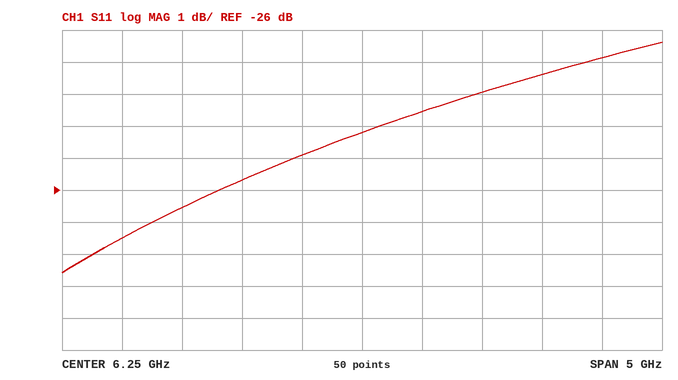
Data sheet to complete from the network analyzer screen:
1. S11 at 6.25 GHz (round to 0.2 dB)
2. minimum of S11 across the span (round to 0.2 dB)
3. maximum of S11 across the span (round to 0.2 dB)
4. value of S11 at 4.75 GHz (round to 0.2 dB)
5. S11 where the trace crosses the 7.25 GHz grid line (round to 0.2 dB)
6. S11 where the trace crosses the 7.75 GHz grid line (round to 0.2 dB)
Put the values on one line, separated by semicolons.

-24.2 dB; -28.6 dB; -21.4 dB; -26.6 dB; -23.0 dB; -22.4 dB
